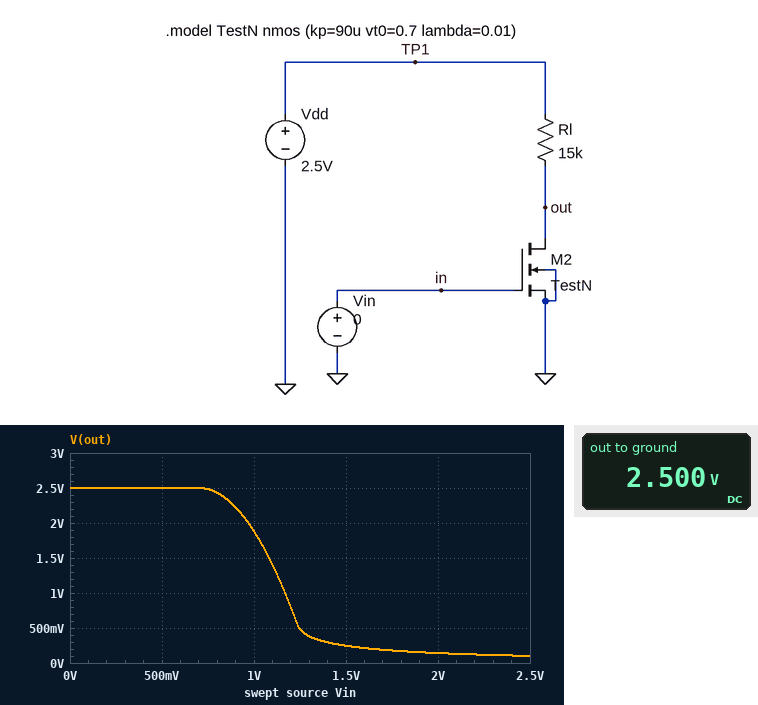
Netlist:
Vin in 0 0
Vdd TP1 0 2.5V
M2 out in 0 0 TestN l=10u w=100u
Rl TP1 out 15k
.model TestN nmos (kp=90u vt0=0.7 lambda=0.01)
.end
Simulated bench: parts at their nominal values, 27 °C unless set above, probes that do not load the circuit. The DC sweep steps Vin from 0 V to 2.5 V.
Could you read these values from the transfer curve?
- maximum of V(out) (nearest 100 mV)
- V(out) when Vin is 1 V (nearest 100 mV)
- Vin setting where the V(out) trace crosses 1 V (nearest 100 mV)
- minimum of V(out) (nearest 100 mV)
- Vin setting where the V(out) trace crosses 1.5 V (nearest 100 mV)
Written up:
2.5 V
1.9 V
1.2 V
100 mV
1.1 V
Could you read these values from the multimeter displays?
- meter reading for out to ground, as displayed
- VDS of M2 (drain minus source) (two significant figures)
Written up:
2.500 V
2.5 V
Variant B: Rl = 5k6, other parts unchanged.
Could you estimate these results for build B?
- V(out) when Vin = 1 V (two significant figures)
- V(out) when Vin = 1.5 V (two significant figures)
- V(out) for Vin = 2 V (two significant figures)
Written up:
2.3 V
870 mV
380 mV
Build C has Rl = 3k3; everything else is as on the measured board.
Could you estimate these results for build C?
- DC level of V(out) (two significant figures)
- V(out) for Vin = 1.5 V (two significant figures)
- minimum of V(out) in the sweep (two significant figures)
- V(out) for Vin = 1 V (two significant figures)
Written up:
2.5 V
1.5 V
440 mV
2.4 V
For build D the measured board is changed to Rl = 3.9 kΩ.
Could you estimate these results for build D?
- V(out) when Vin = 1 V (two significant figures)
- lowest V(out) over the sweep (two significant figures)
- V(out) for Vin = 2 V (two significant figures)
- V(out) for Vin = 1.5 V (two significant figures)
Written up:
2.3 V
370 mV
540 mV
1.4 V
